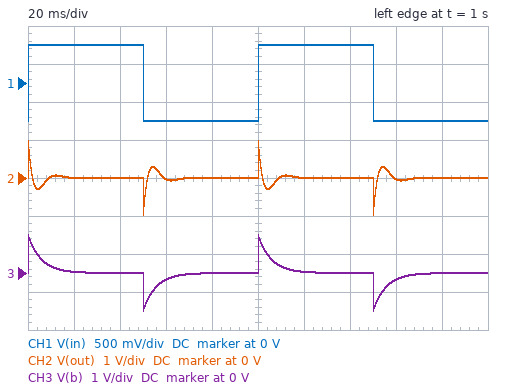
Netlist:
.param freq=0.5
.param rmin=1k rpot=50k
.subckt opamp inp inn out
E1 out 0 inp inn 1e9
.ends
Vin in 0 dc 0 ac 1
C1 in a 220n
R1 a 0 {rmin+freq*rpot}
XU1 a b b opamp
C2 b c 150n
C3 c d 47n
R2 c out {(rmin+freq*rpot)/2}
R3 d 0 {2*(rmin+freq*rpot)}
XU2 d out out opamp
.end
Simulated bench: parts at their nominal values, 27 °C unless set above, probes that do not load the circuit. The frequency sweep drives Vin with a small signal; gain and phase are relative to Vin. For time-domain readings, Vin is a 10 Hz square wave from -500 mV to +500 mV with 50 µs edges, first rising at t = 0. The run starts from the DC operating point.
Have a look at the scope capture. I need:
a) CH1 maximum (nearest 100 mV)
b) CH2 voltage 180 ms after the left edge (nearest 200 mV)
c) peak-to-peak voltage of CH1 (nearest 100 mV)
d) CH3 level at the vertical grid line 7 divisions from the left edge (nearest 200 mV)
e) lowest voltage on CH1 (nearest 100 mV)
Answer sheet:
500 mV
0 V
1.0 V
0 V
-500 mV
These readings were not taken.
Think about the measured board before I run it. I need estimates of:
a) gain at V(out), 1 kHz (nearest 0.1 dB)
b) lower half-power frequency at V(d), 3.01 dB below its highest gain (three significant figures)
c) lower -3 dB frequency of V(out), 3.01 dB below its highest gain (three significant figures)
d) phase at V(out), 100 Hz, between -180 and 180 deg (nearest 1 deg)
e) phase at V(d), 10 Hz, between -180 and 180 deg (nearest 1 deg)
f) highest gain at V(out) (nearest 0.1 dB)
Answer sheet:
0 dB
67.9 Hz
67.9 Hz
77 deg
-119 deg
0.3 dB
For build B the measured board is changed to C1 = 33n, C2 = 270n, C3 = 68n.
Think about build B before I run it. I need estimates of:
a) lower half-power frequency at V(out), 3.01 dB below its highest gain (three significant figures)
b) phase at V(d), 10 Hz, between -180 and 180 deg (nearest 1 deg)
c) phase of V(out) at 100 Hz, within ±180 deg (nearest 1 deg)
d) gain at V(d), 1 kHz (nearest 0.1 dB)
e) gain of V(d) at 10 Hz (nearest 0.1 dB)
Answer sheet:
181 Hz
-109 deg
97 deg
-0.1 dB
-51.5 dB
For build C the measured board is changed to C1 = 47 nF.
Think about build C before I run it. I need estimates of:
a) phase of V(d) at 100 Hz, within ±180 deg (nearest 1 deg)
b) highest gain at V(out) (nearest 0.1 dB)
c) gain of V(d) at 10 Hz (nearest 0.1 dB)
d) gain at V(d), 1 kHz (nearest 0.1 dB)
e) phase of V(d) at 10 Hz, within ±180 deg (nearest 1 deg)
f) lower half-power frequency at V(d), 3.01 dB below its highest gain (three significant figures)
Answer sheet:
114 deg
0 dB
-56.8 dB
-0.1 dB
-104 deg
119 Hz
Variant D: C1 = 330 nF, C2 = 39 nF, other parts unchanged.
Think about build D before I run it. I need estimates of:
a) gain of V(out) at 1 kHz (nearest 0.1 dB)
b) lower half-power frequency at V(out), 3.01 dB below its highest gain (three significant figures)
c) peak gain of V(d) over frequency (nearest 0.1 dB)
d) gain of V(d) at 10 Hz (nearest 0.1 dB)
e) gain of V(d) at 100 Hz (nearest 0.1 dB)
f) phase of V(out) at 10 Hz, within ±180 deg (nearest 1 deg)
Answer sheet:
0.1 dB
123 Hz
1.2 dB
-52.7 dB
-5.1 dB
-122 deg
